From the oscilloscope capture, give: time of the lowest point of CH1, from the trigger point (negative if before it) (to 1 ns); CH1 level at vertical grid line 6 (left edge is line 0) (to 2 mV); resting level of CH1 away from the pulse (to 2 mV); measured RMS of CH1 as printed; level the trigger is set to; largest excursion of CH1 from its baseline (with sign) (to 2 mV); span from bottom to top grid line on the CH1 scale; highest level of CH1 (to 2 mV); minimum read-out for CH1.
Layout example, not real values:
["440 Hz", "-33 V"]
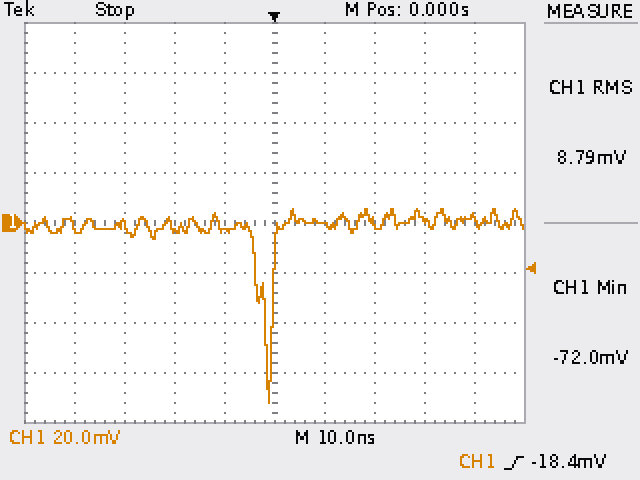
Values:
["-1 ns", "0 mV", "0 mV", "8.79 mV", "-18.4 mV", "-72 mV", "160 mV", "6 mV", "-72.0 mV"]
